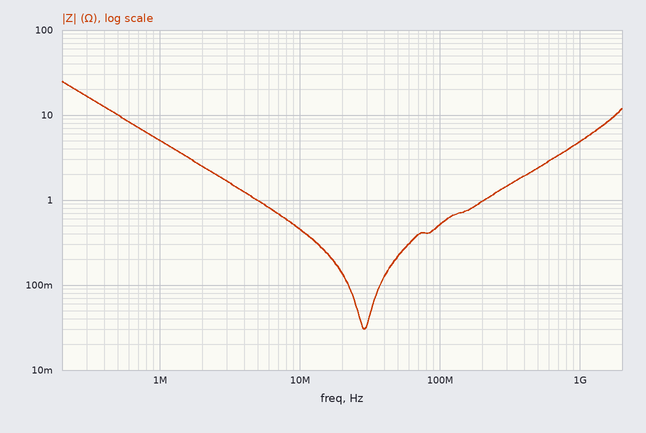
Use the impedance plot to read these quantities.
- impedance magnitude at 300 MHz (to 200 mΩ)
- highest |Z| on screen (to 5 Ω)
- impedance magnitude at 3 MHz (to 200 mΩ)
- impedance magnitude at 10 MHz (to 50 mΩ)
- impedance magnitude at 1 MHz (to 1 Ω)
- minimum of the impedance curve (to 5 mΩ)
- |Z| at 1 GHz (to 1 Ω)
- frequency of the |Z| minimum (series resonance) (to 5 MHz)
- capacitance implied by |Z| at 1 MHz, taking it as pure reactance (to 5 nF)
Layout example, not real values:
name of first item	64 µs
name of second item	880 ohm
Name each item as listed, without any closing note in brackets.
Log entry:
impedance magnitude at 300 MHz	1.4 Ω
highest |Z| on screen	25 Ω
impedance magnitude at 3 MHz	1.6 Ω
impedance magnitude at 10 MHz	450 mΩ
impedance magnitude at 1 MHz	5 Ω
minimum of the impedance curve	30 mΩ
|Z| at 1 GHz	5 Ω
frequency of the |Z| minimum (series resonance)	30 MHz
capacitance implied by |Z| at 1 MHz, taking it as pure reactance	30 nF
